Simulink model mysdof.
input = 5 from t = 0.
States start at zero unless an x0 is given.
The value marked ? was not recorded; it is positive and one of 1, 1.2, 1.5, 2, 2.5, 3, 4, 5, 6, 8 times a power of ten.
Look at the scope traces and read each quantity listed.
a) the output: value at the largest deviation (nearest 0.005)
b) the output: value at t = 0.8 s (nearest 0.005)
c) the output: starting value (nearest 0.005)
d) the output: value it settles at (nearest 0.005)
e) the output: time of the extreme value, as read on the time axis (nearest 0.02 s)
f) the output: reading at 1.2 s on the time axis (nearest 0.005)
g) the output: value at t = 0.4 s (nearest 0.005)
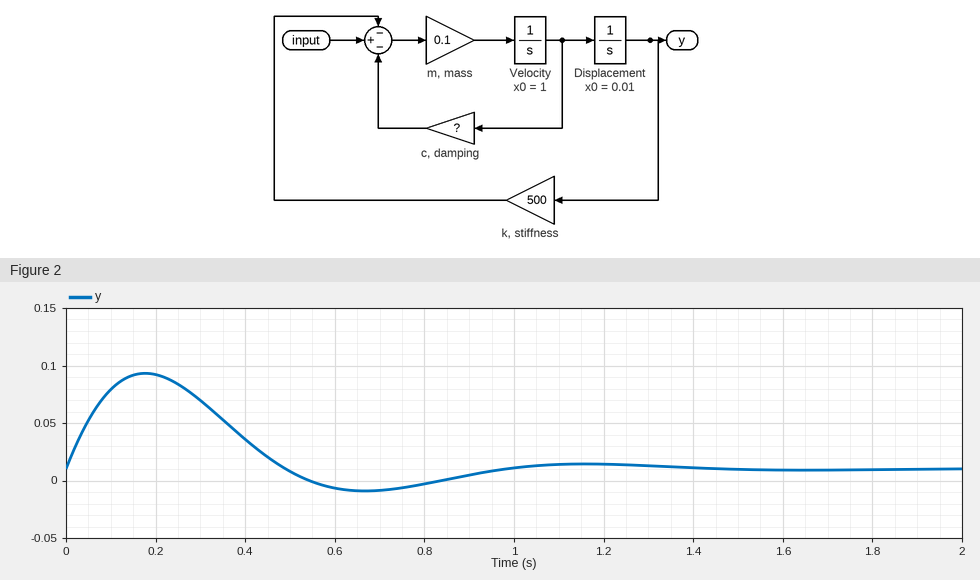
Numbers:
0.095
-0.005
0.010
0.010
0.18 s
0.015
0.035
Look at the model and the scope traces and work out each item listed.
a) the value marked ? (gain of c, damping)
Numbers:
60
